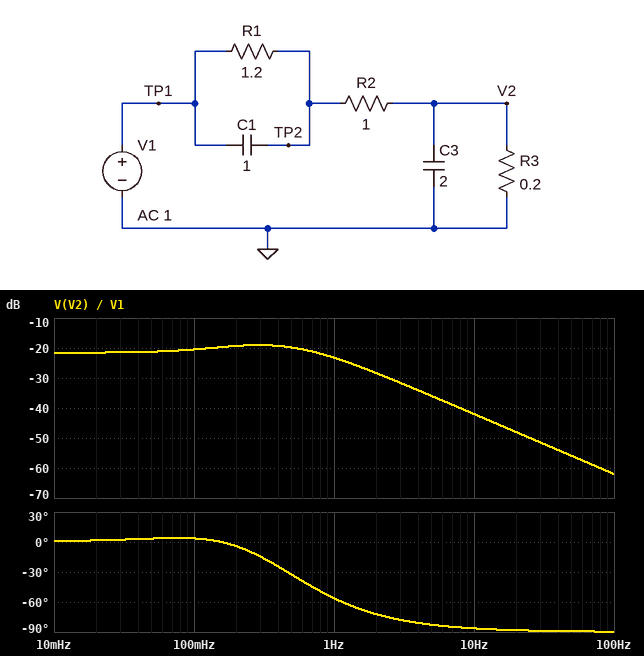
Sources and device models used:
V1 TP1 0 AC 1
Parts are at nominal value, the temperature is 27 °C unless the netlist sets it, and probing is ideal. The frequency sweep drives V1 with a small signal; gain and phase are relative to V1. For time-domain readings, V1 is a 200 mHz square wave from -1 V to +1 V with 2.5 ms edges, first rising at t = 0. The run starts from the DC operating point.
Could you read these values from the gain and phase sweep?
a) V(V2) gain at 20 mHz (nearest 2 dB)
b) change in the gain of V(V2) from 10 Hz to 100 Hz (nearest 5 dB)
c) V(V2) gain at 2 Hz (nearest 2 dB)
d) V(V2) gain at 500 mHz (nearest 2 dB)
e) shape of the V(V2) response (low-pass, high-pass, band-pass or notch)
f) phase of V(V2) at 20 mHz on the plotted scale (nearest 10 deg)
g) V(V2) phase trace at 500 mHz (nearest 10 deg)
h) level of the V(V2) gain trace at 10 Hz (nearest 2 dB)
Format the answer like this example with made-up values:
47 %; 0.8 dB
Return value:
-22 dB; -20 dB; -28 dB; -20 dB; low-pass; 0 deg; -30 deg; -42 dB
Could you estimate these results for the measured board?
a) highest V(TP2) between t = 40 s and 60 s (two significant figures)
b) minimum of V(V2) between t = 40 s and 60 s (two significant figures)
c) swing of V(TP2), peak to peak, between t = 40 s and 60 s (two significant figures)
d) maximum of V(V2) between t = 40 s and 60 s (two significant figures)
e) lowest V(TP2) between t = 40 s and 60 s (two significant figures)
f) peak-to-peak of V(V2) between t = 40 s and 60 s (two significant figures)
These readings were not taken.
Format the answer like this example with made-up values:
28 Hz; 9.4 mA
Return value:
1.5 V; -130 mV; 3.0 V; 130 mV; -1.5 V; 250 mV
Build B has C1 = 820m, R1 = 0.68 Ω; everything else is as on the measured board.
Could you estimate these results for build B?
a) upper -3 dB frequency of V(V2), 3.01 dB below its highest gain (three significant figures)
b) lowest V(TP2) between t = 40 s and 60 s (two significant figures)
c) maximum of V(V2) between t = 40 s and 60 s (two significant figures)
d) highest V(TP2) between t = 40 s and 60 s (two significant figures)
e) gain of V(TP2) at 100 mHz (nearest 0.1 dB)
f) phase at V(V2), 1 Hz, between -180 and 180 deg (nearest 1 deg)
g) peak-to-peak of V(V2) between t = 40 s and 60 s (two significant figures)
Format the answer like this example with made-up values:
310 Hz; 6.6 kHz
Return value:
821 mHz; -1.4 V; 110 mV; 1.4 V; -3.7 dB; -55 deg; 220 mV
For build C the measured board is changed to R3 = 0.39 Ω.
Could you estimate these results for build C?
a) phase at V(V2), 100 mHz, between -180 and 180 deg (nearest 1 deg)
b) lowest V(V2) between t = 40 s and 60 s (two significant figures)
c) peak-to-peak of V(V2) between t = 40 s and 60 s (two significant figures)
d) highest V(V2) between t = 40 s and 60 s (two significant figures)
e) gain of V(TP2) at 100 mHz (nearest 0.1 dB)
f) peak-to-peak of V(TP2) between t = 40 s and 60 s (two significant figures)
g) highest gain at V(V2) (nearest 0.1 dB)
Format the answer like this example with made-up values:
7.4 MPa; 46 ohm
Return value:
-7 deg; -170 mV; 340 mV; 170 mV; -4.4 dB; 2.9 V; -15.8 dB
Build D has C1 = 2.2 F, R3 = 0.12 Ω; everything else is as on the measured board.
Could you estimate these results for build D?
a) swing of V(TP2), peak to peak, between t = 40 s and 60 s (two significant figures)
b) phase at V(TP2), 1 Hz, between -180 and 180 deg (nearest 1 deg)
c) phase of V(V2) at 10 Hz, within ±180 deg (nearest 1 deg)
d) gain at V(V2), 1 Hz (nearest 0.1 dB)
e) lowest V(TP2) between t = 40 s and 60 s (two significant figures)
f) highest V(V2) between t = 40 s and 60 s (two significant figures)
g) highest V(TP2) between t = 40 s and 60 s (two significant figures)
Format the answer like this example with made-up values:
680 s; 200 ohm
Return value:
2.8 V; 4 deg; -85 deg; -24.0 dB; -1.4 V; 110 mV; 1.4 V
